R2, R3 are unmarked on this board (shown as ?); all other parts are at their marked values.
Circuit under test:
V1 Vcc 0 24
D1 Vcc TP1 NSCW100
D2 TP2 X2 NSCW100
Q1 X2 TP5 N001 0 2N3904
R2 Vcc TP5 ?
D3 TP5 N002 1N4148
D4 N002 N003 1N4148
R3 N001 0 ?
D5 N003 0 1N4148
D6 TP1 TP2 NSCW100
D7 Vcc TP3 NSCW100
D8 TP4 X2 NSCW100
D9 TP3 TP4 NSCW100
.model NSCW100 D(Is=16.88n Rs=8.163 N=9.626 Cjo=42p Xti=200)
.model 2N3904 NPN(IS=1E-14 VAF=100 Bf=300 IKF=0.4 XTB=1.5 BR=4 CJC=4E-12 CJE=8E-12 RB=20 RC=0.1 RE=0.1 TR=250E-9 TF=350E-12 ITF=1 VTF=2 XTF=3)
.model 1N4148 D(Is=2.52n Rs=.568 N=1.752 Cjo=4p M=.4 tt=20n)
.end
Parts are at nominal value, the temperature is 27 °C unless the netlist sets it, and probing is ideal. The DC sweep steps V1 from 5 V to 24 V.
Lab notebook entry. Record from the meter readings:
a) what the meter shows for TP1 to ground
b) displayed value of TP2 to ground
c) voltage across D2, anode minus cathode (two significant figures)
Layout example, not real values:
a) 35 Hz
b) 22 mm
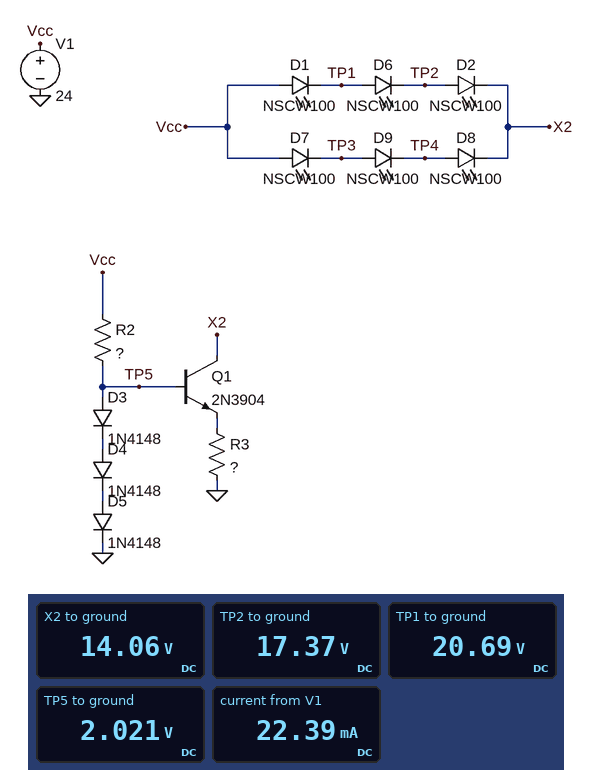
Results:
a) 20.69 V
b) 17.37 V
c) 3.3 V
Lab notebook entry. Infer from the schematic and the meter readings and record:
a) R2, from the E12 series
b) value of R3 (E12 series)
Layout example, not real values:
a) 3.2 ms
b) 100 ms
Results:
a) 3.3 kΩ
b) 82 Ω
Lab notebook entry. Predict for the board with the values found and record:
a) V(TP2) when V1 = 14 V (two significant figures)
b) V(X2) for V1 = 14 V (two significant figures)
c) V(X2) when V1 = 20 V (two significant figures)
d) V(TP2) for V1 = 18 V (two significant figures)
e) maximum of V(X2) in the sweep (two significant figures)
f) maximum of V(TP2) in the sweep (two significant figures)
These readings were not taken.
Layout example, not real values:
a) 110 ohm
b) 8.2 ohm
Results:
a) 7.4 V
b) 4.1 V
c) 10 V
d) 11 V
e) 14 V
f) 17 V
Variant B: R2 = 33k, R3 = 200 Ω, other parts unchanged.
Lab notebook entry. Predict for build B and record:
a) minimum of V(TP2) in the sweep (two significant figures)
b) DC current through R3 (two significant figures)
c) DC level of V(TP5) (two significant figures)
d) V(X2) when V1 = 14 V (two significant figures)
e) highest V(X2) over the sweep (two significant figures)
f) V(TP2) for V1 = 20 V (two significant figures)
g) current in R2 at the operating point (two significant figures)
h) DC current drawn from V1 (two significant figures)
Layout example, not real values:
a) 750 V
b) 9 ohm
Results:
a) 1.7 V
b) 5.0 mA
c) 1.7 V
d) 5.1 V
e) 15 V
f) 14 V
g) 680 µA
h) 5.7 mA
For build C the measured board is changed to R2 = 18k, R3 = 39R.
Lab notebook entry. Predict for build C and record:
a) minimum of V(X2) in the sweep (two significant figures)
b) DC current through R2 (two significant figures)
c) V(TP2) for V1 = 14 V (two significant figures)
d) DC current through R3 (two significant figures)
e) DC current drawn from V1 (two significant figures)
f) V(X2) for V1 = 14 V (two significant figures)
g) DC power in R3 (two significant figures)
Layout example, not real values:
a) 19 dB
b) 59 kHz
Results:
a) 17 mV
b) 1.2 mA
c) 7.1 V
d) 26 mA
e) 28 mA
f) 3.6 V
g) 27 mW
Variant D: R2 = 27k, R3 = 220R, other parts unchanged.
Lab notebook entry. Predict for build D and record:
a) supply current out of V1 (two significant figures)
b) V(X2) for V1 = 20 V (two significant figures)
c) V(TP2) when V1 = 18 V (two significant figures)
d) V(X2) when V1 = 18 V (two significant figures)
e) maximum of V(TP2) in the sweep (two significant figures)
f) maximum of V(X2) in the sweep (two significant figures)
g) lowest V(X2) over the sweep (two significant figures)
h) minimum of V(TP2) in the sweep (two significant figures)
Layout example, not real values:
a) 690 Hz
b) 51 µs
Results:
a) 5.5 mA
b) 11 V
c) 12 V
d) 9.1 V
e) 18 V
f) 15 V
g) 47 mV
h) 1.7 V
